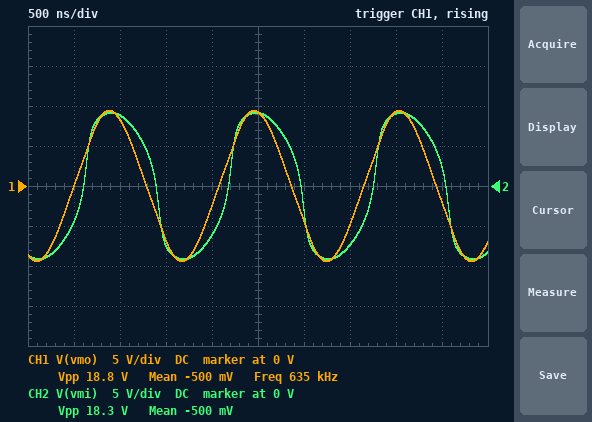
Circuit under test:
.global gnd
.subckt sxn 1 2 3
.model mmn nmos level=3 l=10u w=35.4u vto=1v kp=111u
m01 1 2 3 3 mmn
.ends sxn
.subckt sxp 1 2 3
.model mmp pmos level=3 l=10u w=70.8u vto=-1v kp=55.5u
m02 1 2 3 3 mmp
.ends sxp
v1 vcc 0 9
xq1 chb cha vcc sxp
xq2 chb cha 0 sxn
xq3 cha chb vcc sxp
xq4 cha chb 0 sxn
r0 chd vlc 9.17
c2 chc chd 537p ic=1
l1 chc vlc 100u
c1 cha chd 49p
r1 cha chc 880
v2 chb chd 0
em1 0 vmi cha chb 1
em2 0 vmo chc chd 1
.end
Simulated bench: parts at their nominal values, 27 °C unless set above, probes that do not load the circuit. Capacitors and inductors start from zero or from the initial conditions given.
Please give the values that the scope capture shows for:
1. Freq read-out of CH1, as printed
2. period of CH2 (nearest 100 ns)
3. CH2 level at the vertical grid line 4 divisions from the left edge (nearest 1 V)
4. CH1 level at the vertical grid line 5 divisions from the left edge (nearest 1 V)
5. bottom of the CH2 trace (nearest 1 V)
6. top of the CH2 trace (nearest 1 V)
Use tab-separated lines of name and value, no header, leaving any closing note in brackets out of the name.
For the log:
Freq read-out of CH1, as printed	635 kHz
period of CH2	1.6 µs
CH2 level at the vertical grid line 4 divisions from the left edge	-6 V
CH1 level at the vertical grid line 5 divisions from the left edge	9 V
bottom of the CH2 trace	-9 V
top of the CH2 trace	9 V
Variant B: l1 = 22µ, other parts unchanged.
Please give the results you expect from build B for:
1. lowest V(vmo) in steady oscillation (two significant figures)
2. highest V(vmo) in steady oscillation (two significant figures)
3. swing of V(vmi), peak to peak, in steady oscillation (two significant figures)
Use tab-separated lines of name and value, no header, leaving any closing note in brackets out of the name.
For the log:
lowest V(vmo) in steady oscillation	-710 mV
highest V(vmo) in steady oscillation	650 mV
swing of V(vmi), peak to peak, in steady oscillation	3.1 V
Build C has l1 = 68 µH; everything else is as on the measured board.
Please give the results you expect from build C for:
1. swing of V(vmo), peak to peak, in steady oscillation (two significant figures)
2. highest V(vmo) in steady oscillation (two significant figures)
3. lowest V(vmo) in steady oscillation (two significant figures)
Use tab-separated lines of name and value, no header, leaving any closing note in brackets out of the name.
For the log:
swing of V(vmo), peak to peak, in steady oscillation	17 V
highest V(vmo) in steady oscillation	8.6 V
lowest V(vmo) in steady oscillation	-8.6 V
